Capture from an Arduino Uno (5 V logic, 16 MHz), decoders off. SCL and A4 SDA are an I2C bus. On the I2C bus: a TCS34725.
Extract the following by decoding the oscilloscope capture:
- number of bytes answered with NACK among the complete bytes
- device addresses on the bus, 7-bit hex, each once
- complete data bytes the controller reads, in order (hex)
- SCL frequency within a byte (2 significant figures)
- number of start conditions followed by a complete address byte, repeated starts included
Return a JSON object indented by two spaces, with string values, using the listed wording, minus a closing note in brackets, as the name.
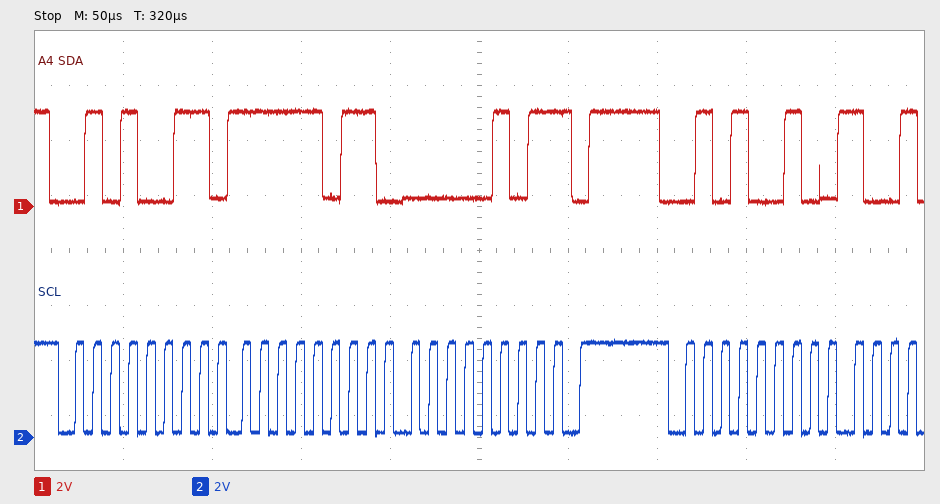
{
  "number of bytes answered with NACK among the complete bytes": "1",
  "device addresses on the bus, 7-bit hex, each once": "0x29",
  "complete data bytes the controller reads, in order": "FB 05",
  "SCL frequency within a byte": "100 kHz",
  "number of start conditions followed by a complete address byte, repeated starts included": "2"
}
